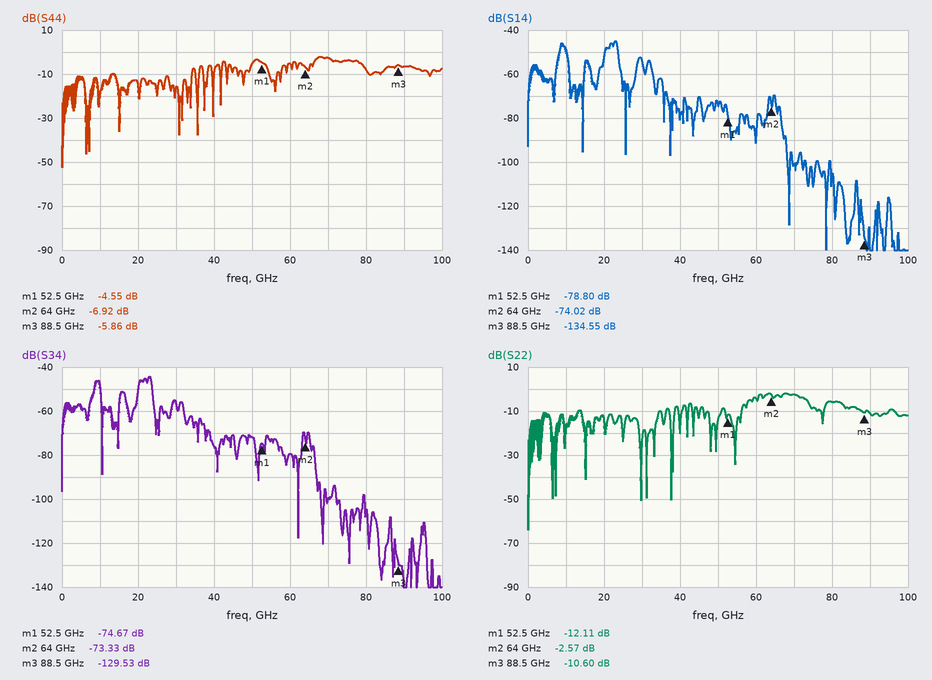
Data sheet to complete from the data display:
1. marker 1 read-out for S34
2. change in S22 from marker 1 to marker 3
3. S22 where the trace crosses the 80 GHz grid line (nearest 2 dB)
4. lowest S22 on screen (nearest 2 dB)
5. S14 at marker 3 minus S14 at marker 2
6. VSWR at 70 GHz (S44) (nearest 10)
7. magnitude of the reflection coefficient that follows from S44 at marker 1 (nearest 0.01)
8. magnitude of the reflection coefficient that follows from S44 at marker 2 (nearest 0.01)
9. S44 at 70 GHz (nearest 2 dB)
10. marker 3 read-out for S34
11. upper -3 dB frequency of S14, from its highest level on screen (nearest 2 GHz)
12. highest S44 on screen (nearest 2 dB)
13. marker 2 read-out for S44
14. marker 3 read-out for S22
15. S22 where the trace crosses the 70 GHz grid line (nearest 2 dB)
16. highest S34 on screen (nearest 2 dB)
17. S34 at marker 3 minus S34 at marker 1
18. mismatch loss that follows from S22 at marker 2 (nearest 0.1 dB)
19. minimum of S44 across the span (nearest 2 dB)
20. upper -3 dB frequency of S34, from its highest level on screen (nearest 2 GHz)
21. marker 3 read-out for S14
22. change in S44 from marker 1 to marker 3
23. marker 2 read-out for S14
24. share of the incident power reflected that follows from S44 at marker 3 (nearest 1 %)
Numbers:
-74.67 dB
1.51 dB
-6 dB
-64 dB
-60.53 dB
10
0.59
0.45
-2 dB
-129.53 dB
24 GHz
-2 dB
-6.92 dB
-10.60 dB
-2 dB
-44 dB
-54.86 dB
3.5 dB
-52 dB
24 GHz
-134.55 dB
-1.31 dB
-74.02 dB
26 %
